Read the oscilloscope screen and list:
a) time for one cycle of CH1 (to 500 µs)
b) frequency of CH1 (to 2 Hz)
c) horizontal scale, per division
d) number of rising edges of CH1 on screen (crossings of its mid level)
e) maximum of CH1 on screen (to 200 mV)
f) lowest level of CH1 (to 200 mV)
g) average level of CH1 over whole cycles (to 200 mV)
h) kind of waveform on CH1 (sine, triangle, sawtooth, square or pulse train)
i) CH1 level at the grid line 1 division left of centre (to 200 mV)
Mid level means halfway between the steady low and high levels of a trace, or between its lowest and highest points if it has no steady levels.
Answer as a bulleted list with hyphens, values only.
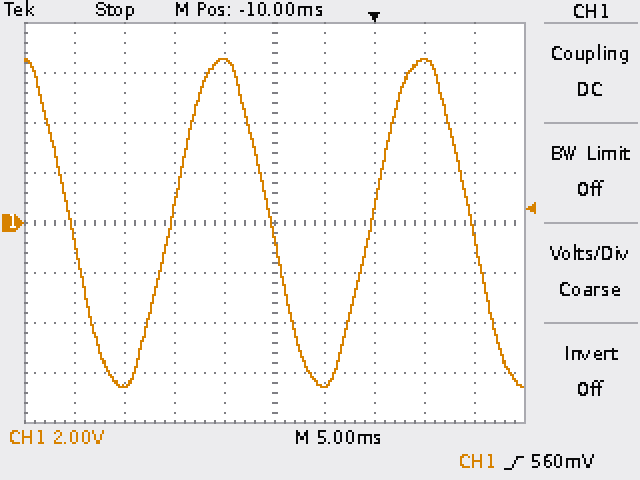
- 20.0 ms
- 50 Hz
- 5 ms
- 2
- 6.6 V
- -6.6 V
- 0.0 V
- sine
- 6.6 V
